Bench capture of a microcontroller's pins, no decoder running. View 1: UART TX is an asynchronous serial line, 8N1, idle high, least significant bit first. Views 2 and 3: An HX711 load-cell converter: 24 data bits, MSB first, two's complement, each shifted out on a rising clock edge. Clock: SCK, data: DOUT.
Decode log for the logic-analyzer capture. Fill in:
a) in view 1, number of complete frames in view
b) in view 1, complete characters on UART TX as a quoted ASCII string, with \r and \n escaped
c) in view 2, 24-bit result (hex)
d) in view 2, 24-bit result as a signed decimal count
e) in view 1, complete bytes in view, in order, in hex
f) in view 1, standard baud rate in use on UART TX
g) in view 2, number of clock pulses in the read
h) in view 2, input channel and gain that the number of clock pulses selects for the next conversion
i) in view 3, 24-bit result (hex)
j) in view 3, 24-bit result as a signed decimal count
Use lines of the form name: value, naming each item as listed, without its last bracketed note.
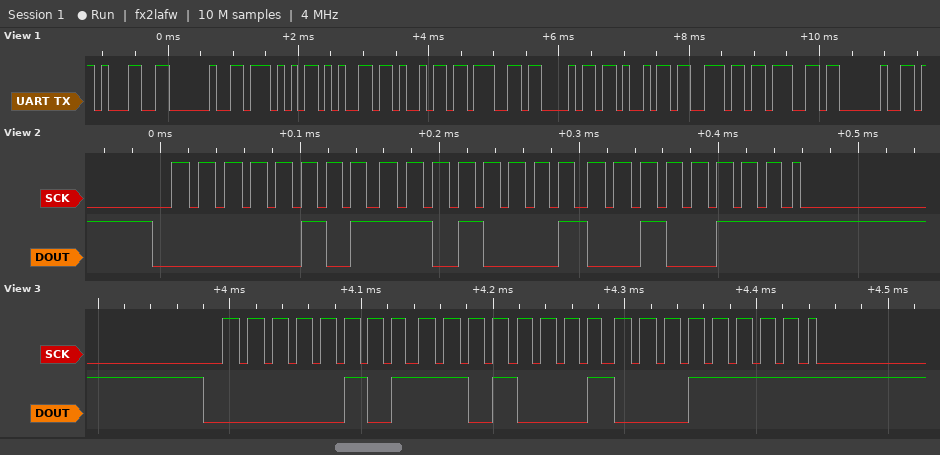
in view 1, number of complete frames in view: 11
in view 1, complete characters on UART TX as a quoted ASCII string, with \r and \n escaped: "1 Weighing "
in view 2, 24-bit result: 0x05D127
in view 2, 24-bit result as a signed decimal count: 381223
in view 1, complete bytes in view, in order, in hex: 31 20 57 65 69 67 68 69 6E 67 20
in view 1, standard baud rate in use on UART TX: 9600 baud
in view 2, number of clock pulses in the read: 25
in view 2, input channel and gain that the number of clock pulses selects for the next conversion: channel A, gain 128
in view 3, 24-bit result: 0x05D11F
in view 3, 24-bit result as a signed decimal count: 381215
